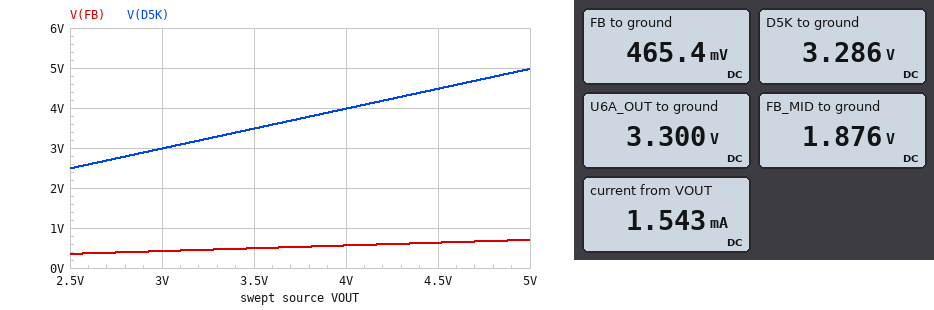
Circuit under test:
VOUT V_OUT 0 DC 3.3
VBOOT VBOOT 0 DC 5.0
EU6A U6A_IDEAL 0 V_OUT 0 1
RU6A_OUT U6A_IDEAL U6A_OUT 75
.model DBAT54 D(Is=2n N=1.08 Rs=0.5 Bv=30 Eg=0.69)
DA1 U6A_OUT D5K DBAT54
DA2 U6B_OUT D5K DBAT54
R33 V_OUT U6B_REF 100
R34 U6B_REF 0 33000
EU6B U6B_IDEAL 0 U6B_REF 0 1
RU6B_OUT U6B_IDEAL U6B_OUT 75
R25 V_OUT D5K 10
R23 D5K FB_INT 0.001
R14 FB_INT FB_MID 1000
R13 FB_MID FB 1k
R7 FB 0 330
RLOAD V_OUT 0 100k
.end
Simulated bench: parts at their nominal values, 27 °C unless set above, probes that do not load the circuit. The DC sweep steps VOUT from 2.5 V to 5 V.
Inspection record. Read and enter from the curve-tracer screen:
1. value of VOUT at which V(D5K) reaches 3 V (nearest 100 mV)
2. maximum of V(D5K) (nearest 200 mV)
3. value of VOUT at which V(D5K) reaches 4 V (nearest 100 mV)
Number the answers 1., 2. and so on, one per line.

1. 3.0 V
2. 5.0 V
3. 4.0 V
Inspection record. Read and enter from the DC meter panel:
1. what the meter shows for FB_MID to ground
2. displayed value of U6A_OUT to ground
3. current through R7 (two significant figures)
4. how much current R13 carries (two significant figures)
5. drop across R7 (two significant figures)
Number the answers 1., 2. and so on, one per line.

1. 1.876 V
2. 3.300 V
3. 1.4 mA
4. 1.4 mA
5. 470 mV
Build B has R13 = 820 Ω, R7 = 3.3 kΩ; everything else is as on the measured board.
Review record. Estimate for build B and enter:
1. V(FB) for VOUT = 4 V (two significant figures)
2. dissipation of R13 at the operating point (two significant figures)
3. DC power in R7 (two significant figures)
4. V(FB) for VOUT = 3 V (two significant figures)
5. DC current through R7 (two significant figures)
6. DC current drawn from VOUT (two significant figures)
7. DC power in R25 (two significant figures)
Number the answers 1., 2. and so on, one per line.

1. 2.6 V
2. 340 µW
3. 1.4 mW
4. 1.9 V
5. 640 µA
6. 780 µA
7. 4.1 µW
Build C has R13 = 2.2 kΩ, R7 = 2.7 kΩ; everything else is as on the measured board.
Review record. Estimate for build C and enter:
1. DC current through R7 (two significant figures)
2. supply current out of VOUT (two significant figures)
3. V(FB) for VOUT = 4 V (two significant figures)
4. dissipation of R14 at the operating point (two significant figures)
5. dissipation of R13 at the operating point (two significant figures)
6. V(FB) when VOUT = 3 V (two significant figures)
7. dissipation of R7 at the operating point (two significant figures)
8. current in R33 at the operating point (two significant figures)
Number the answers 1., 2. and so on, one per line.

1. 560 µA
2. 690 µA
3. 1.8 V
4. 310 µW
5. 690 µW
6. 1.4 V
7. 840 µW
8. 100 µA
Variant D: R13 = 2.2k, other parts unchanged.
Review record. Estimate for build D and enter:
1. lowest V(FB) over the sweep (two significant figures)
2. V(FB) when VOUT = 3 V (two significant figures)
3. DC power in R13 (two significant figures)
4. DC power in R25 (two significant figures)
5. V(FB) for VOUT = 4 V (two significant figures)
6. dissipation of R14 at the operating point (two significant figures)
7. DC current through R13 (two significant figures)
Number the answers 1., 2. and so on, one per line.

1. 230 mV
2. 280 mV
3. 1.9 mW
4. 8.7 µW
5. 370 mV
6. 870 µW
7. 930 µA
